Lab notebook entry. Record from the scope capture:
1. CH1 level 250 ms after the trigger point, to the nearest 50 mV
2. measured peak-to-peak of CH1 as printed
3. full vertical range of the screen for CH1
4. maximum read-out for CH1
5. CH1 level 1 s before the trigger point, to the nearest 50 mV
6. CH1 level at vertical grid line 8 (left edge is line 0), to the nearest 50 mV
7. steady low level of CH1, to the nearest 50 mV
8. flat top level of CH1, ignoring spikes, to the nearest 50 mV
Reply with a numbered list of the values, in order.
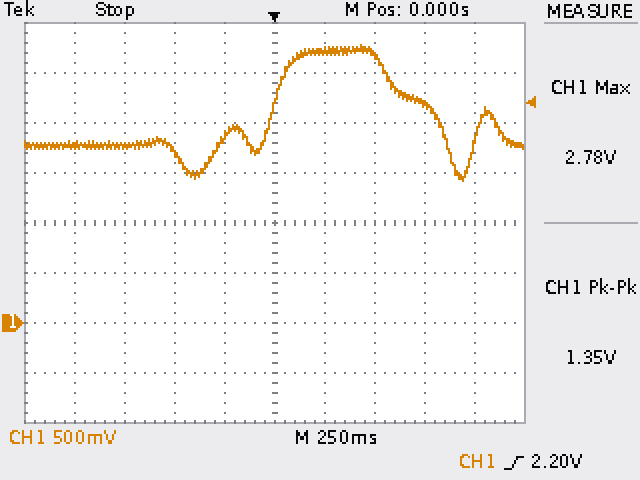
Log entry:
1. 2.70 V
2. 1.35 V
3. 4 V
4. 2.78 V
5. 1.80 V
6. 2.20 V
7. 1.80 V
8. 2.70 V
